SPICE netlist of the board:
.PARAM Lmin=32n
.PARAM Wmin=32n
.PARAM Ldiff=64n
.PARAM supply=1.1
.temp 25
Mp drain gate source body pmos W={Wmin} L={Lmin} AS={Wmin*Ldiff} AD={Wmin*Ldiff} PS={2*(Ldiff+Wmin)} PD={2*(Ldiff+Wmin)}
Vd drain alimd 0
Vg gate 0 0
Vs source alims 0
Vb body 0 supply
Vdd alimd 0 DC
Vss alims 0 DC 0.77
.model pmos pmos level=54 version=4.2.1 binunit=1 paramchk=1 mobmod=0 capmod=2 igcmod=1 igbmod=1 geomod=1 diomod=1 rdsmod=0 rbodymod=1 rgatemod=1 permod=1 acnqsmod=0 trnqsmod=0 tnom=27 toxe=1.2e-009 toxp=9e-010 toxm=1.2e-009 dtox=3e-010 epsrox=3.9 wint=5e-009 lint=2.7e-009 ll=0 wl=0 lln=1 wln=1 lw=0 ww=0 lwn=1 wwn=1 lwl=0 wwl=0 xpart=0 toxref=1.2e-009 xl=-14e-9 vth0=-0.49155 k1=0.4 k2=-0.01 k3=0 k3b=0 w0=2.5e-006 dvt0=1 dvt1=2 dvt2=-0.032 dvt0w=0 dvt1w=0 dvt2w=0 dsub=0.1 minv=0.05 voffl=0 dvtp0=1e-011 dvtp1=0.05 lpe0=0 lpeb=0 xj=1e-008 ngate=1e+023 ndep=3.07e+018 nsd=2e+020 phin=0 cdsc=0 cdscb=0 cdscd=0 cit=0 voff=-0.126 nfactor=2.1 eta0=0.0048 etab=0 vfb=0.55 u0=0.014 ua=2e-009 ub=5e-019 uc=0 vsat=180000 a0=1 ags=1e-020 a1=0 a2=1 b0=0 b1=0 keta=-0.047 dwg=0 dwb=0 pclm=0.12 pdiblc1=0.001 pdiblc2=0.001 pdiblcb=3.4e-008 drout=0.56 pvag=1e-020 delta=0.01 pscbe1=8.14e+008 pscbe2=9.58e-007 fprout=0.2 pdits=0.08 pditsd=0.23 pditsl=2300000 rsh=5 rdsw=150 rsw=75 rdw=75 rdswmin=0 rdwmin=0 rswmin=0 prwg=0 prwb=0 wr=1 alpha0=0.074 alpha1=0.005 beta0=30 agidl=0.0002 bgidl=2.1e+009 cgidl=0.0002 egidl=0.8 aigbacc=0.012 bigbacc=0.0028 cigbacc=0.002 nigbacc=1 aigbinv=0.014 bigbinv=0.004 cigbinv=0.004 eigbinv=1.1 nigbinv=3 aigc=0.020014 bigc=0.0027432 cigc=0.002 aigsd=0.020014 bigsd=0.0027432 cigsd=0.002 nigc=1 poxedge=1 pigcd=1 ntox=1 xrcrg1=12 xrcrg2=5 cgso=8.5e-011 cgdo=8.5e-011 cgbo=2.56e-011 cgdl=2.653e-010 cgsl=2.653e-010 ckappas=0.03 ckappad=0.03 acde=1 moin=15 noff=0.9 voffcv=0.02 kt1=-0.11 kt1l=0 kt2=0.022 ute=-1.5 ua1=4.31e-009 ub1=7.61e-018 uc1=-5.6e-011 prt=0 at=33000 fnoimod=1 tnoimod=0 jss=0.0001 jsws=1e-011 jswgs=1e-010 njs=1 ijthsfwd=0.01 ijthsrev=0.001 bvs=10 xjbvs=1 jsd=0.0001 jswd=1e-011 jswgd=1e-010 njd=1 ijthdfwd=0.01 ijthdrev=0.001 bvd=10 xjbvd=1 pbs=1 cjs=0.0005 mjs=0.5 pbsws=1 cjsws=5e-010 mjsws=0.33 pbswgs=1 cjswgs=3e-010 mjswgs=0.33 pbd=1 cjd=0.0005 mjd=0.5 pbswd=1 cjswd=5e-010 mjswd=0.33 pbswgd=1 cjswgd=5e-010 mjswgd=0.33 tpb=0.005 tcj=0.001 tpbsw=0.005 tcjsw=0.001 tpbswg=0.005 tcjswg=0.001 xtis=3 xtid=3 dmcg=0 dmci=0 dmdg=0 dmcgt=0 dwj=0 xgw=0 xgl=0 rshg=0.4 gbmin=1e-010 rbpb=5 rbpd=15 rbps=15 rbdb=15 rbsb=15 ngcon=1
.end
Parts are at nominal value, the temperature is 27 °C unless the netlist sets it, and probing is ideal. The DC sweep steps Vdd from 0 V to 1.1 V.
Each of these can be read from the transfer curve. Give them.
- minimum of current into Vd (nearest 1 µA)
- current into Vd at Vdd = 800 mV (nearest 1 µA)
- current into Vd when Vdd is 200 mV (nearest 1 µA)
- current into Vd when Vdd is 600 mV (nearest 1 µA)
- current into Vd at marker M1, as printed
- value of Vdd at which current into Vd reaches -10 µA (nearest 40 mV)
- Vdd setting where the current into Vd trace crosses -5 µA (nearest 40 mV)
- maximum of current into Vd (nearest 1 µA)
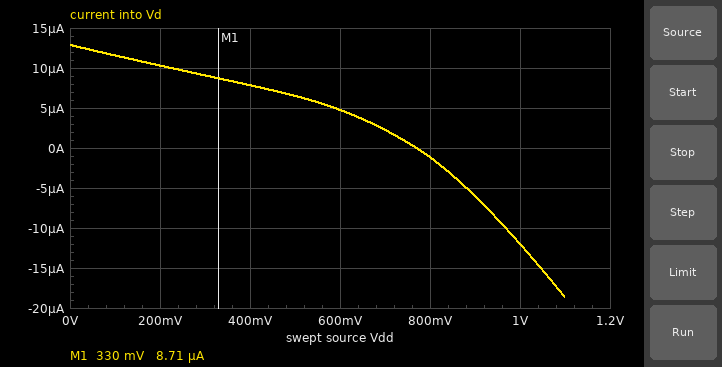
-19 µA
-1 µA
10 µA
5 µA
8.71 µA
960 mV
880 mV
13 µA
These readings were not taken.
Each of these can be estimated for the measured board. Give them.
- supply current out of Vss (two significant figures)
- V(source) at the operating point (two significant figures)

13 µA
770 mV
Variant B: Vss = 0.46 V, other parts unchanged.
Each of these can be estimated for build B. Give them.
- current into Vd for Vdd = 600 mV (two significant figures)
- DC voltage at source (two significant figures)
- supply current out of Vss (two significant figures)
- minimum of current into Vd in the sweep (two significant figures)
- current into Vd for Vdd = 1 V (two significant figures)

-800 nA
460 mV
180 nA
-28 µA
-21 µA
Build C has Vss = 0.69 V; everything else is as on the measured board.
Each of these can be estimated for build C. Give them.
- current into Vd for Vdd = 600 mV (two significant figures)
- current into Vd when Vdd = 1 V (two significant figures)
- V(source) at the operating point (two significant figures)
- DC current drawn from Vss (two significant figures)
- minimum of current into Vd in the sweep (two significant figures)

1.7 µA
-15 µA
690 mV
7.9 µA
-22 µA
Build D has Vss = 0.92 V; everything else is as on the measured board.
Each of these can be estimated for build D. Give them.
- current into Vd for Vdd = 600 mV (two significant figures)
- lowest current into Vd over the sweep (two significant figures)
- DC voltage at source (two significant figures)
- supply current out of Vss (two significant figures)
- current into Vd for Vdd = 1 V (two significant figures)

13 µA
-11 µA
920 mV
23 µA
-4.7 µA
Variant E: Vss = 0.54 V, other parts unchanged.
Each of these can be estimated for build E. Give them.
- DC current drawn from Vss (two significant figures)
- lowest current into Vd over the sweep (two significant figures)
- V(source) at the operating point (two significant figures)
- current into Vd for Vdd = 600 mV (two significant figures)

1.3 µA
-26 µA
540 mV
-440 nA
